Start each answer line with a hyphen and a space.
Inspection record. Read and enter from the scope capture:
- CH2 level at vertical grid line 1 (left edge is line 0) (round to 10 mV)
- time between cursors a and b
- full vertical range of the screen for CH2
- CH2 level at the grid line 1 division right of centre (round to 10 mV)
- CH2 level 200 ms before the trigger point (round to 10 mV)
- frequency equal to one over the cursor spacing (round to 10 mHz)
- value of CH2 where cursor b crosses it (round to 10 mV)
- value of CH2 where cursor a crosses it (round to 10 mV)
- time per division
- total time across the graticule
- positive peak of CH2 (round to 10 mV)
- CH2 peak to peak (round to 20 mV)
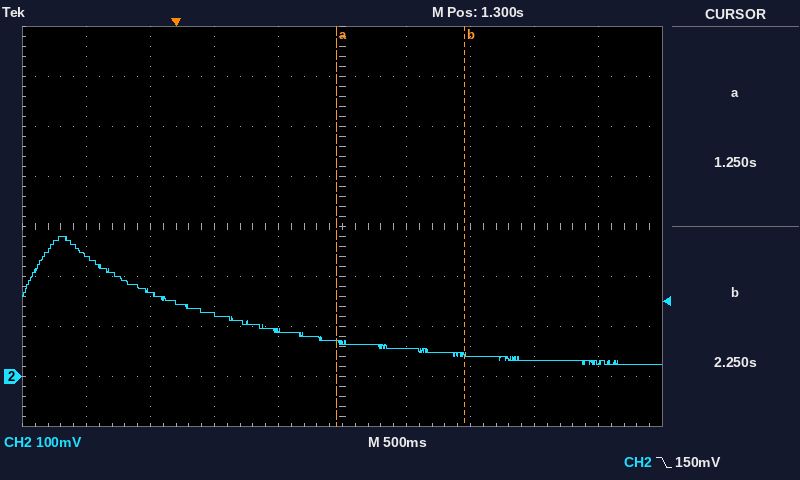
- 240 mV
- 1.00 s
- 800 mV
- 60 mV
- 170 mV
- 1.00 Hz
- 40 mV
- 70 mV
- 500 ms
- 5 s
- 280 mV
- 260 mV
